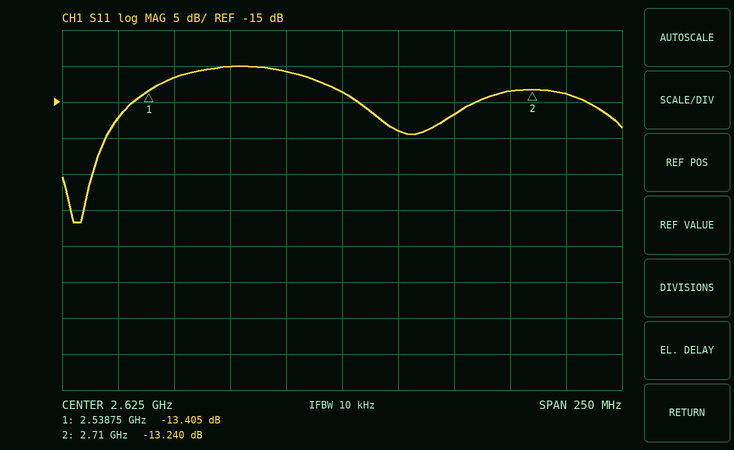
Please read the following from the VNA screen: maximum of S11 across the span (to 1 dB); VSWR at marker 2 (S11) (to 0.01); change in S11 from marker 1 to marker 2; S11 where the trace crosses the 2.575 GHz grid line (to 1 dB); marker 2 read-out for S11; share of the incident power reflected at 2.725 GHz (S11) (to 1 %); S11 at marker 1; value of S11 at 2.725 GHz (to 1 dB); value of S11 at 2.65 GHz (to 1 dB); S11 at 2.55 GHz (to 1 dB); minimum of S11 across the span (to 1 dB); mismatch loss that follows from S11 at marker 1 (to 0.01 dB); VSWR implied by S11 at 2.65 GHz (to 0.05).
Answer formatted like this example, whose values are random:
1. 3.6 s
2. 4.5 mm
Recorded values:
1. -10 dB
2. 1.56
3. 0.165 dB
4. -10 dB
5. -13.240 dB
6. 4 %
7. -13.405 dB
8. -14 dB
9. -19 dB
10. -12 dB
11. -32 dB
12. 0.20 dB
13. 1.25
